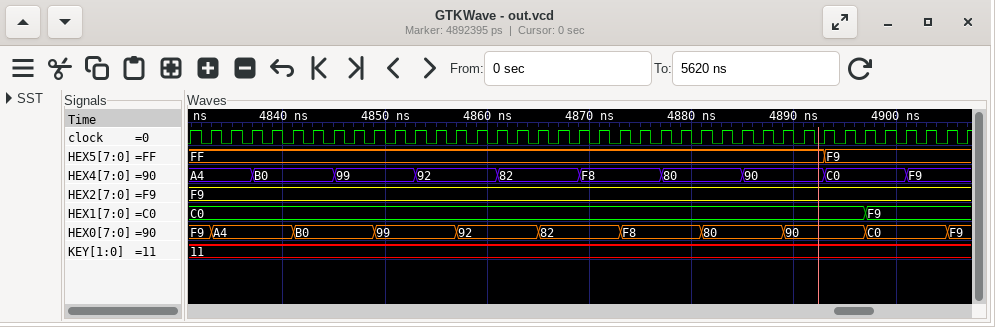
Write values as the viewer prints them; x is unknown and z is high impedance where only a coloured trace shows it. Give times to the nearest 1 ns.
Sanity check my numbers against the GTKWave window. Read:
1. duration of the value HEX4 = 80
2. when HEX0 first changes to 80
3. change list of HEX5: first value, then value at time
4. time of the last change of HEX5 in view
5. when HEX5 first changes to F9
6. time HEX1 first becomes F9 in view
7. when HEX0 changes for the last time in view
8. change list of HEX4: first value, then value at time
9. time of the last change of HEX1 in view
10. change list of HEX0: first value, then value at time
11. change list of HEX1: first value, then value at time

8 ns
4881 ns
FF, F9 at 4893 ns
4893 ns
4893 ns
4897 ns
4905 ns
A4, B0 at 4837 ns, 99 at 4845 ns, 92 at 4853 ns, 82 at 4861 ns, F8 at 4869 ns, 80 at 4877 ns, 90 at 4885 ns, C0 at 4893 ns, F9 at 4901 ns
4897 ns
F9, A4 at 4833 ns, B0 at 4841 ns, 99 at 4849 ns, 92 at 4857 ns, 82 at 4865 ns, F8 at 4873 ns, 80 at 4881 ns, 90 at 4889 ns, C0 at 4897 ns, F9 at 4905 ns
C0, F9 at 4897 ns
